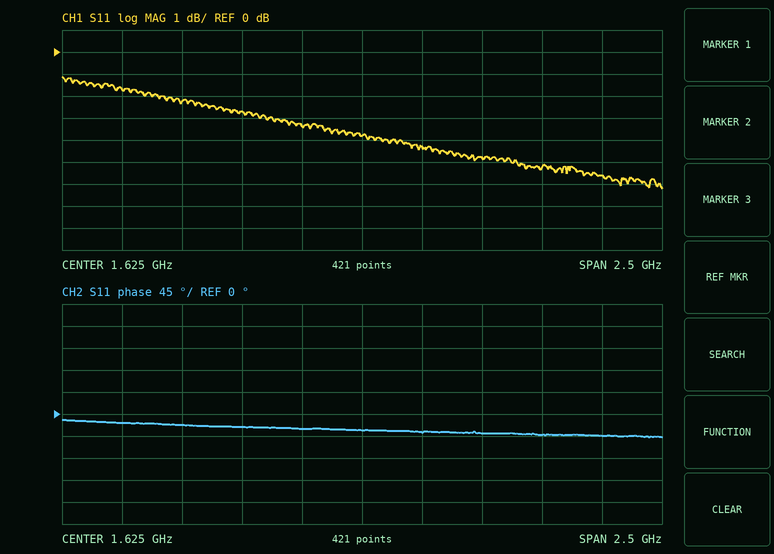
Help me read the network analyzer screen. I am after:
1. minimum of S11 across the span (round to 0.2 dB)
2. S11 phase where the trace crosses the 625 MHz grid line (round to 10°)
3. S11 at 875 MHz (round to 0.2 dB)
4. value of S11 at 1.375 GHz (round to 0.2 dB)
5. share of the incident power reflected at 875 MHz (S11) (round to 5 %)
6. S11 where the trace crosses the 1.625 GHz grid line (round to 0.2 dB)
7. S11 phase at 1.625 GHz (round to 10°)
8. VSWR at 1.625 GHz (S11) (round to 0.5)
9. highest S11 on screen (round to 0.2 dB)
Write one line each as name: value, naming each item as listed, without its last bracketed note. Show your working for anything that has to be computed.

minimum of S11 across the span: -6.2 dB
S11 phase where the trace crosses the 625 MHz grid line: -20°
S11 at 875 MHz: -2.2 dB
value of S11 at 1.375 GHz: -3.4 dB
share of the incident power reflected at 875 MHz (S11): 10^(-2.2/10) ≈ 60 %
S11 where the trace crosses the 1.625 GHz grid line: -3.8 dB
S11 phase at 1.625 GHz: -30°
VSWR at 1.625 GHz (S11): |Γ| = 10^(-3.8/20) = 0.6457; VSWR = (1 + 0.6457)/(1 − 0.6457) ≈ 4.64, so 4.5 to the nearest 0.5
highest S11 on screen: -1.2 dB
